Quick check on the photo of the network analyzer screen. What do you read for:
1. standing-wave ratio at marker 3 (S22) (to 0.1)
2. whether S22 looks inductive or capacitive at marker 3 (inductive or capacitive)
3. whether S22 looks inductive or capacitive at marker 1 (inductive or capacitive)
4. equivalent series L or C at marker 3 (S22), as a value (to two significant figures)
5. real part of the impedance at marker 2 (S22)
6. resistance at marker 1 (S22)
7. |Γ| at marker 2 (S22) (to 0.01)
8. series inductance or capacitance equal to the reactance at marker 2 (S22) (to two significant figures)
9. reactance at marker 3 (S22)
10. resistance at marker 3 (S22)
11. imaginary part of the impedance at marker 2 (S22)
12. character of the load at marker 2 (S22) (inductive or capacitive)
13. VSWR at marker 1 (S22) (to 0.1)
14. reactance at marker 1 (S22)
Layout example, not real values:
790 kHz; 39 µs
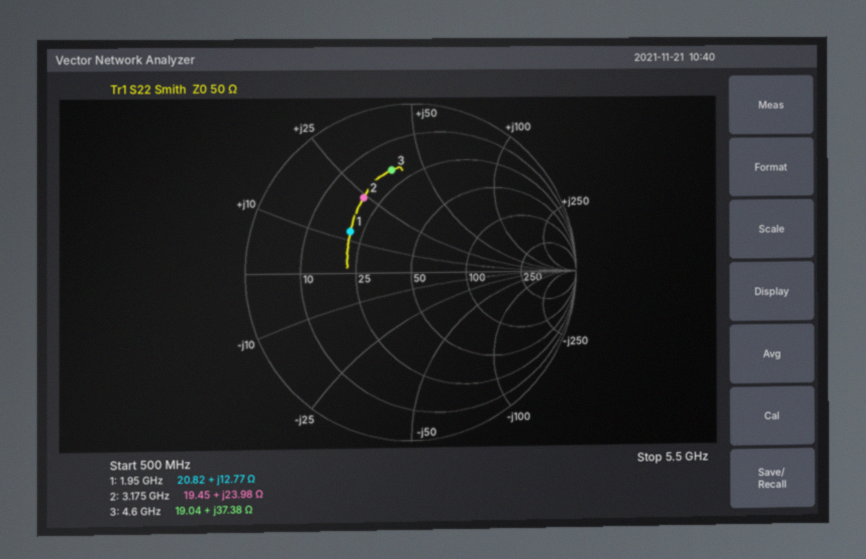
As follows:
4.2; inductive; inductive; 1.3 nH; 19.45 Ω; 20.82 Ω; 0.53; 1.2 nH; +37.38 Ω; 19.04 Ω; +23.98 Ω; inductive; 2.6; +12.77 Ω
